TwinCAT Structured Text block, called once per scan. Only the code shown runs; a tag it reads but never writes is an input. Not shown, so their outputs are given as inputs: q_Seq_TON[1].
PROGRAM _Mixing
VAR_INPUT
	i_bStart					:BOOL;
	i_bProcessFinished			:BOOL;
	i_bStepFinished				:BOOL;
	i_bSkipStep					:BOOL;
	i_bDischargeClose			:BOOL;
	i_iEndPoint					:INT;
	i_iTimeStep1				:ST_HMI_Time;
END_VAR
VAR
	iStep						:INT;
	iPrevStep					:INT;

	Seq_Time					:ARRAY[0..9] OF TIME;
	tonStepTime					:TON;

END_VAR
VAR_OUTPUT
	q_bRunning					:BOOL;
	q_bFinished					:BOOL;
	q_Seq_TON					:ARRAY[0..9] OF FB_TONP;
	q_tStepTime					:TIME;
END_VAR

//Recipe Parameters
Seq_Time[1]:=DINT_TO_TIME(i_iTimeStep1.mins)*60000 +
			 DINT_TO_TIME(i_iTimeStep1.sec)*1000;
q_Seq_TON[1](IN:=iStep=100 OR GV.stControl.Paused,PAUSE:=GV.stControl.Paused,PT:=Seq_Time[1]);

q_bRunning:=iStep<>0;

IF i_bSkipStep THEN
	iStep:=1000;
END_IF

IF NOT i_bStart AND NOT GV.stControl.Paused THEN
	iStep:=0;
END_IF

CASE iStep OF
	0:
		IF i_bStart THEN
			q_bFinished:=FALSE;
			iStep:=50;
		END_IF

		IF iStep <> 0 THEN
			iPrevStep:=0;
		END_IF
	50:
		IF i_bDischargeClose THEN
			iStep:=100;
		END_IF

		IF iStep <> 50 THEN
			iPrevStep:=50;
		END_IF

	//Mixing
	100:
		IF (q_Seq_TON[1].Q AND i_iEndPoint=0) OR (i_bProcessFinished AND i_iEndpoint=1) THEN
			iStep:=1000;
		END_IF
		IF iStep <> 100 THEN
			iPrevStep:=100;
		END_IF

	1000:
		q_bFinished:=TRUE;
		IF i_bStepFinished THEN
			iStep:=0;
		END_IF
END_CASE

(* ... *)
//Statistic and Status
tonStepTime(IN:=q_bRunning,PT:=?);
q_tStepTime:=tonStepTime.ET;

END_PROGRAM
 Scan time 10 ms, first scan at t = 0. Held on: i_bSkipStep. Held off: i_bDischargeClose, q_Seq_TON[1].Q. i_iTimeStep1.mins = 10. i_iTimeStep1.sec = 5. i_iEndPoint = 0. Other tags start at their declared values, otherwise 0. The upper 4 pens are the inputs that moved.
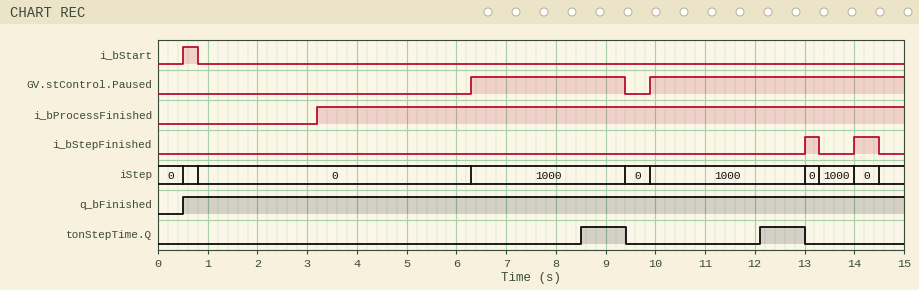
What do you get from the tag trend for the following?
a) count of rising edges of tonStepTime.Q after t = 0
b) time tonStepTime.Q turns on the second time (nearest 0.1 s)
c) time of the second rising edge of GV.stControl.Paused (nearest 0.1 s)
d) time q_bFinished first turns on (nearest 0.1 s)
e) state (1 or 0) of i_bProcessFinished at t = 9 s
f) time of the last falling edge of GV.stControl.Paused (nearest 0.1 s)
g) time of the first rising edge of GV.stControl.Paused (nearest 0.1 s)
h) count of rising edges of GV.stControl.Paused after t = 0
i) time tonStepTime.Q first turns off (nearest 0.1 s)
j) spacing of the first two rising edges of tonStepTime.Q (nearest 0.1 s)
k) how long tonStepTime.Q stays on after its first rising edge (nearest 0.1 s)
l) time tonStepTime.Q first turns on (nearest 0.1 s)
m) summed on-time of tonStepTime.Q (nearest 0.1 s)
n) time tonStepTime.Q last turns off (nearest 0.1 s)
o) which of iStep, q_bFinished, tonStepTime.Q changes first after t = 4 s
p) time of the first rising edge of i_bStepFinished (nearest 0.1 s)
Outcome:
2
12.1 s
9.9 s
0.5 s
1
9.4 s
6.3 s
2
9.4 s
3.6 s
0.9 s
8.5 s
1.8 s
13.0 s
iStep
13.0 s
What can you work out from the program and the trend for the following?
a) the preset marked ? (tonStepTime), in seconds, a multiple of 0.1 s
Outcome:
2.2 s
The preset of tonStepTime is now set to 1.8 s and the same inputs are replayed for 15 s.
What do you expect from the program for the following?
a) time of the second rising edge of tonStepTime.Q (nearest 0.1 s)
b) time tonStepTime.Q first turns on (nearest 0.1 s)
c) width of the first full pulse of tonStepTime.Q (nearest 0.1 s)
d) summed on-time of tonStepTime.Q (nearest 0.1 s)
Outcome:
11.7 s
8.1 s
1.3 s
2.6 s
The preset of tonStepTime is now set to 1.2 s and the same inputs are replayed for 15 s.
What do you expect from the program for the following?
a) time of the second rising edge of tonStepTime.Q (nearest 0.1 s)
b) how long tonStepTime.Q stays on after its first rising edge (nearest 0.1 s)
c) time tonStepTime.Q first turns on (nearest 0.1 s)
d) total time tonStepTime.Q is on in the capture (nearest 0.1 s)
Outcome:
11.1 s
1.9 s
7.5 s
3.8 s
